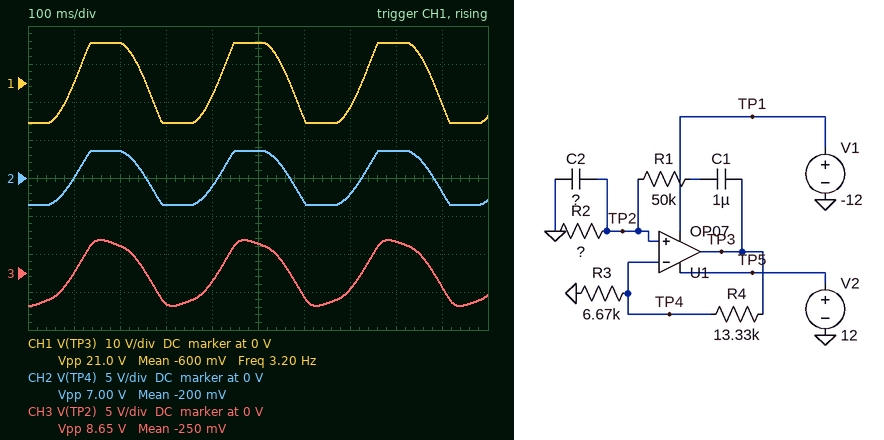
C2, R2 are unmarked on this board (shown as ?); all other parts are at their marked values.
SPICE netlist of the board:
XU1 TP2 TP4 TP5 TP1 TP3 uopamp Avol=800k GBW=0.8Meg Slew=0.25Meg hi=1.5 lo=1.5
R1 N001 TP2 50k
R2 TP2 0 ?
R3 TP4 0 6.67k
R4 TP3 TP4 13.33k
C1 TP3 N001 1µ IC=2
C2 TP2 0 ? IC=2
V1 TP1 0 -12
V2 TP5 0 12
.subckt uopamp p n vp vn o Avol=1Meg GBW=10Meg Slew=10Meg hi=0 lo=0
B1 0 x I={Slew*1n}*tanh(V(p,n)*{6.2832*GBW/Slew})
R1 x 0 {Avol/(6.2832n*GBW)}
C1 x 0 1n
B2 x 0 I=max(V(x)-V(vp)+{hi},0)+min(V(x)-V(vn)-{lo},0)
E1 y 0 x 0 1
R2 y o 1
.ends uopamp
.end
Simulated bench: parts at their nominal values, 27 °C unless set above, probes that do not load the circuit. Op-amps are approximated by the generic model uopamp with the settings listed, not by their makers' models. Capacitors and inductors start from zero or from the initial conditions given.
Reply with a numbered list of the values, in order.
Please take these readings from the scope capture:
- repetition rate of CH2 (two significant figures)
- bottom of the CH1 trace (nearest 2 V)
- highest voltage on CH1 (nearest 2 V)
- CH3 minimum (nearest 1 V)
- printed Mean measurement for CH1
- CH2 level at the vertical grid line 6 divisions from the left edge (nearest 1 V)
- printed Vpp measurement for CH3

1. 3.2 Hz
2. -10 V
3. 10 V
4. -4 V
5. -600 mV
6. -3 V
7. 8.65 V
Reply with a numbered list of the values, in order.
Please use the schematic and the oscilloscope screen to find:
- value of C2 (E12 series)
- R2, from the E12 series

1. 820 nF
2. 56 kΩ
